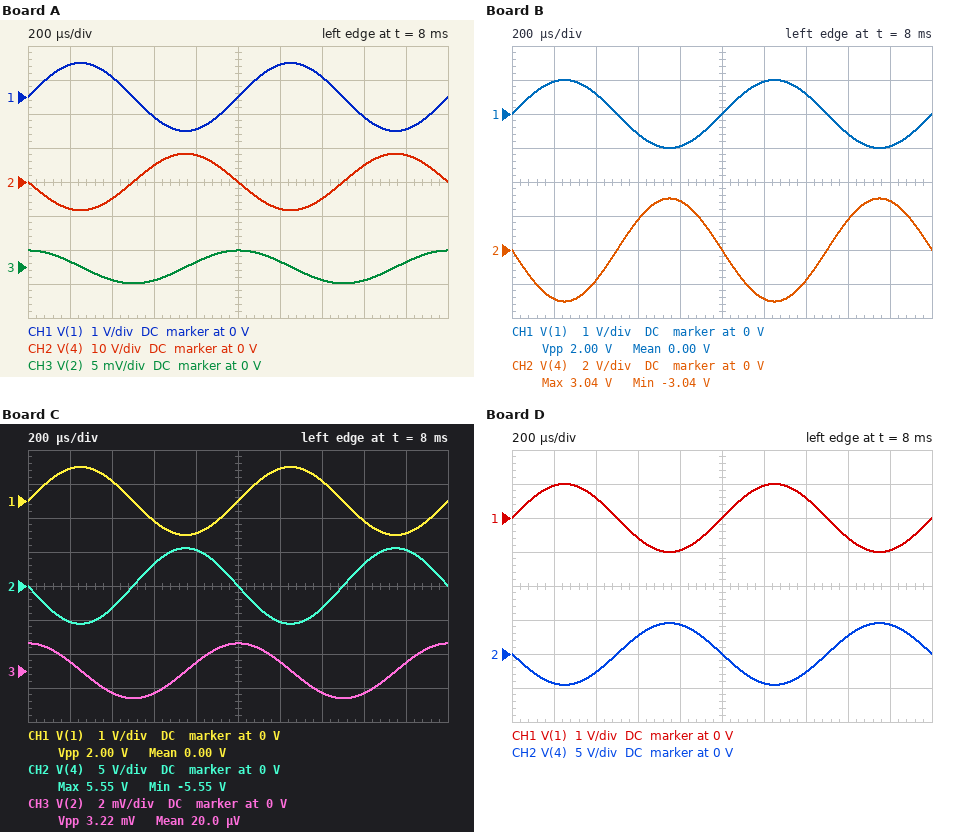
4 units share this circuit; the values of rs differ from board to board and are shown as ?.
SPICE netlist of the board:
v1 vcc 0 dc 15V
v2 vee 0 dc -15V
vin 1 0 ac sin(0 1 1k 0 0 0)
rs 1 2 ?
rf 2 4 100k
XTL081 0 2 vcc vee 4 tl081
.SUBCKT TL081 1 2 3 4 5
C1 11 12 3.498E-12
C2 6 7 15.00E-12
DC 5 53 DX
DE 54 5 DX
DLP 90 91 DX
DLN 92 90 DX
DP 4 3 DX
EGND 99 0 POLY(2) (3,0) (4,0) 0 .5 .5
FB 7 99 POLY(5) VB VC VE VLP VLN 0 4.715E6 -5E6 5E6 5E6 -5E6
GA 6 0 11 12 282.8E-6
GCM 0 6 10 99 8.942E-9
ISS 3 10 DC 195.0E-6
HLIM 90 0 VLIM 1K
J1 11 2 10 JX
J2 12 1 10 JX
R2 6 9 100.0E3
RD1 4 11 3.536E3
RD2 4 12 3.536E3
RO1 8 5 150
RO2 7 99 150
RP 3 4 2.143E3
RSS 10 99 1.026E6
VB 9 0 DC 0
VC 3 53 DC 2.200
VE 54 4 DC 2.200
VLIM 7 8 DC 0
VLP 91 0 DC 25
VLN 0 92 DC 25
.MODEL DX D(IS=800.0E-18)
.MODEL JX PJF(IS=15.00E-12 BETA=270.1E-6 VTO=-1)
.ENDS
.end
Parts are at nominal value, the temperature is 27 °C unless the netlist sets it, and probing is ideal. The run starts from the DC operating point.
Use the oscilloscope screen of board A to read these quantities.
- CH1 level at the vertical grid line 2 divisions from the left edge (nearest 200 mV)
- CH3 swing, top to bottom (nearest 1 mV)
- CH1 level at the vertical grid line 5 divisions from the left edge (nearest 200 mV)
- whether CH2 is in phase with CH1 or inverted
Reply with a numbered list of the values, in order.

1. 600 mV
2. 5 mV
3. 0 V
4. inverted
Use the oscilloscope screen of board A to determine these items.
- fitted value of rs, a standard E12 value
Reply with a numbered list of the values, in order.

1. 12 kΩ
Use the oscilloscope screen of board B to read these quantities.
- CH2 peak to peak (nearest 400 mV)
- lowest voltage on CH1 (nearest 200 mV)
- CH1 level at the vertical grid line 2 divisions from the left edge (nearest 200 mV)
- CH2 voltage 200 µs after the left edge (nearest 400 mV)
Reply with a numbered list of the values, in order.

1. 6.0 V
2. -1.0 V
3. 600 mV
4. -2.8 V
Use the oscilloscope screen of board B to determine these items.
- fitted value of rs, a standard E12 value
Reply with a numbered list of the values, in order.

1. 33 kΩ
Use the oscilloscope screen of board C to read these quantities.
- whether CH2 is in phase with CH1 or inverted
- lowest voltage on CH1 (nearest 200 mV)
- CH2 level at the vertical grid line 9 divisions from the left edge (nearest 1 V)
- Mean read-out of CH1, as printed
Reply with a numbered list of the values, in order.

1. inverted
2. -1.0 V
3. 5 V
4. 0.00 V
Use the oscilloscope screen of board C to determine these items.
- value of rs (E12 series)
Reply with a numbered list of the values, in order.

1. 18 kΩ
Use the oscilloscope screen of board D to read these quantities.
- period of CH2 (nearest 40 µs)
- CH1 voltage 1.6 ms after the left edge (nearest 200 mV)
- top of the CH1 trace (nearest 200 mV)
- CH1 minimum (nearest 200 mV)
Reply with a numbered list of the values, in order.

1. 1.00 ms
2. -600 mV
3. 1.0 V
4. -1.0 V
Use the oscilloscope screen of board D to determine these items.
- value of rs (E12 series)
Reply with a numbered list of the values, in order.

1. 22 kΩ
